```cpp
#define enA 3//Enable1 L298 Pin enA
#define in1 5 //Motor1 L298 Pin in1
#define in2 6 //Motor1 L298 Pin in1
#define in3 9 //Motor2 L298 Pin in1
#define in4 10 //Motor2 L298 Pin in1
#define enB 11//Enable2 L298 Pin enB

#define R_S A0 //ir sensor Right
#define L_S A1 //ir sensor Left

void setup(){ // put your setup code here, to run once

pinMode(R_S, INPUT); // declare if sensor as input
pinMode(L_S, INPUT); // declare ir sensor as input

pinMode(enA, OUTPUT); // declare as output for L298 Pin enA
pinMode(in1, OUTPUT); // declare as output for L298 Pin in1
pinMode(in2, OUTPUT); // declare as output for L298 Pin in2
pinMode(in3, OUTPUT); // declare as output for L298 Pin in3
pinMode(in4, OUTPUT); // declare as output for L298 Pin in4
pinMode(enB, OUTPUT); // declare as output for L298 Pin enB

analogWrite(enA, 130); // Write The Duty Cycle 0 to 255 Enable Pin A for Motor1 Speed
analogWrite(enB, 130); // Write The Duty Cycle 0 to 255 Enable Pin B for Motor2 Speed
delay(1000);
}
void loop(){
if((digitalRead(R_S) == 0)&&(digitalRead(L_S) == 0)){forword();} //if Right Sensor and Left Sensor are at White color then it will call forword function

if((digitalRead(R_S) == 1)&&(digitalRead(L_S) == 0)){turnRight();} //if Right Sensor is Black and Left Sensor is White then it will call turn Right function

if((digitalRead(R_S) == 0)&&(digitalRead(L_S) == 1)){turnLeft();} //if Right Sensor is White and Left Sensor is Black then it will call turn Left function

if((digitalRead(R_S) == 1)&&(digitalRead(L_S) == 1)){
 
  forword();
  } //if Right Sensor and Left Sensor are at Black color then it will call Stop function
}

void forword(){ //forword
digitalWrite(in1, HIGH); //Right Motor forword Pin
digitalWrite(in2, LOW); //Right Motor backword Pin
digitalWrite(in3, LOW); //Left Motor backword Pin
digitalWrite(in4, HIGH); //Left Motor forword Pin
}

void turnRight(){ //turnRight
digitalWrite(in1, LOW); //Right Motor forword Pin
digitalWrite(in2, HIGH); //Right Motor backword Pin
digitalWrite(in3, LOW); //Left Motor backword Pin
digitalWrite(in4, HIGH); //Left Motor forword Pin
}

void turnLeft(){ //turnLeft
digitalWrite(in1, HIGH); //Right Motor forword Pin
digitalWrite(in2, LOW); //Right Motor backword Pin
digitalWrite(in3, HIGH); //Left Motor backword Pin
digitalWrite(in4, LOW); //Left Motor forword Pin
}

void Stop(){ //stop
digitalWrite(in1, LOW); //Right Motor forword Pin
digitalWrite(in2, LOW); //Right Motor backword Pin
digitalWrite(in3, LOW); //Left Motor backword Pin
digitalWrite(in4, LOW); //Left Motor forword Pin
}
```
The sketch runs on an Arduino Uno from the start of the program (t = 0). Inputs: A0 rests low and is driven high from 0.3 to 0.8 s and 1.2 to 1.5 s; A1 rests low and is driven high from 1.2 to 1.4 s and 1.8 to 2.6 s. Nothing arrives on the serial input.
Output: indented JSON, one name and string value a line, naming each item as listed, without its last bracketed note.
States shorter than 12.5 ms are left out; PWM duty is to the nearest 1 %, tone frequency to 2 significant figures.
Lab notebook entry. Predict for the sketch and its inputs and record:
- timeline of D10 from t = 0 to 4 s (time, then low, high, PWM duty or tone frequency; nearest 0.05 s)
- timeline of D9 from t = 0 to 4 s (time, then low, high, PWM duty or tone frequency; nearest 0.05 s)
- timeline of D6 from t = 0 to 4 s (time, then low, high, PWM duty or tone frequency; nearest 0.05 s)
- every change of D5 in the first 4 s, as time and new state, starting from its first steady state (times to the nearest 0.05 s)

{
  "timeline of D10 from t = 0 to 4 s": "0 s low; 1 s high; 1.8 s low; 2.6 s high",
  "timeline of D9 from t = 0 to 4 s": "0 s low; 1.8 s high; 2.6 s low",
  "timeline of D6 from t = 0 to 4 s": "0 s low; 1.4 s high; 1.5 s low",
  "every change of D5 in the first 4 s, as time and new state, starting from its first steady state": "0 s low; 1 s high; 1.4 s low; 1.5 s high"
}
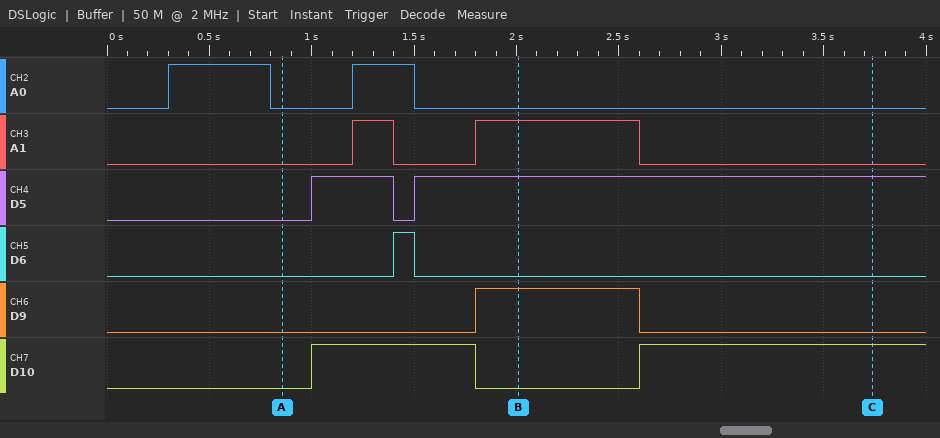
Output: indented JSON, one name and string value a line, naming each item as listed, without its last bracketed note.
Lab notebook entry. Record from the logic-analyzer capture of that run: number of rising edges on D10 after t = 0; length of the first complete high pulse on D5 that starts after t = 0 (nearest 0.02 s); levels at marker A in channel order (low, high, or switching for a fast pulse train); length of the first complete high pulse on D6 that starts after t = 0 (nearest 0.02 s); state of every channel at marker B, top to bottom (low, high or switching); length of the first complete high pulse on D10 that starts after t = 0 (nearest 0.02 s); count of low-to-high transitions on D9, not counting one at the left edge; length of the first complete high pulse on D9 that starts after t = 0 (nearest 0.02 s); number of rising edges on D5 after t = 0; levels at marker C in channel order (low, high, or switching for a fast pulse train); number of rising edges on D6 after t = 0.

{
  "number of rising edges on D10 after t = 0": "2",
  "length of the first complete high pulse on D5 that starts after t = 0": "0.40 s",
  "levels at marker A in channel order": "A0 low, A1 low, D5 low, D6 low, D9 low, D10 low",
  "length of the first complete high pulse on D6 that starts after t = 0": "0.10 s",
  "state of every channel at marker B, top to bottom": "A0 low, A1 high, D5 high, D6 low, D9 high, D10 low",
  "length of the first complete high pulse on D10 that starts after t = 0": "0.80 s",
  "count of low-to-high transitions on D9, not counting one at the left edge": "1",
  "length of the first complete high pulse on D9 that starts after t = 0": "0.80 s",
  "number of rising edges on D5 after t = 0": "2",
  "levels at marker C in channel order": "A0 low, A1 low, D5 high, D6 low, D9 low, D10 high",
  "number of rising edges on D6 after t = 0": "1"
}
